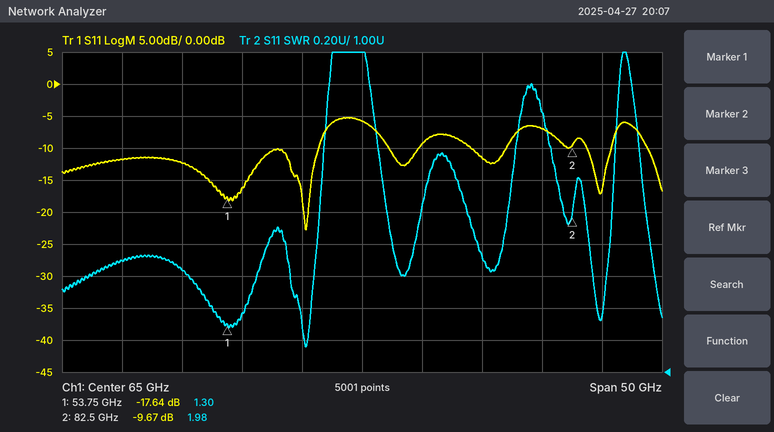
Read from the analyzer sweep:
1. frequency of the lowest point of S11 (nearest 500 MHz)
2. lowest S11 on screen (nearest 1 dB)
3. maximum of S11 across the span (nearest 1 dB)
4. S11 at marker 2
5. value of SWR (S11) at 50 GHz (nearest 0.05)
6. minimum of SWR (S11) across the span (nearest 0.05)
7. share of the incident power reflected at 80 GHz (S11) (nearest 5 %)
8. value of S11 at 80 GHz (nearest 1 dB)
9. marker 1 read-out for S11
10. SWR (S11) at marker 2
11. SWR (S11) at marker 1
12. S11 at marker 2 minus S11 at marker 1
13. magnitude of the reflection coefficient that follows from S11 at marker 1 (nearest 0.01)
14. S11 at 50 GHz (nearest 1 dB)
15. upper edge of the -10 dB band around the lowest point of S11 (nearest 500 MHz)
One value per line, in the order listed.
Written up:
60.5 GHz
-23 dB
-5 dB
-9.67 dB
1.65
1.15
20 %
-7 dB
-17.64 dB
1.98
1.30
7.97 dB
0.13
-12 dB
61.5 GHz
